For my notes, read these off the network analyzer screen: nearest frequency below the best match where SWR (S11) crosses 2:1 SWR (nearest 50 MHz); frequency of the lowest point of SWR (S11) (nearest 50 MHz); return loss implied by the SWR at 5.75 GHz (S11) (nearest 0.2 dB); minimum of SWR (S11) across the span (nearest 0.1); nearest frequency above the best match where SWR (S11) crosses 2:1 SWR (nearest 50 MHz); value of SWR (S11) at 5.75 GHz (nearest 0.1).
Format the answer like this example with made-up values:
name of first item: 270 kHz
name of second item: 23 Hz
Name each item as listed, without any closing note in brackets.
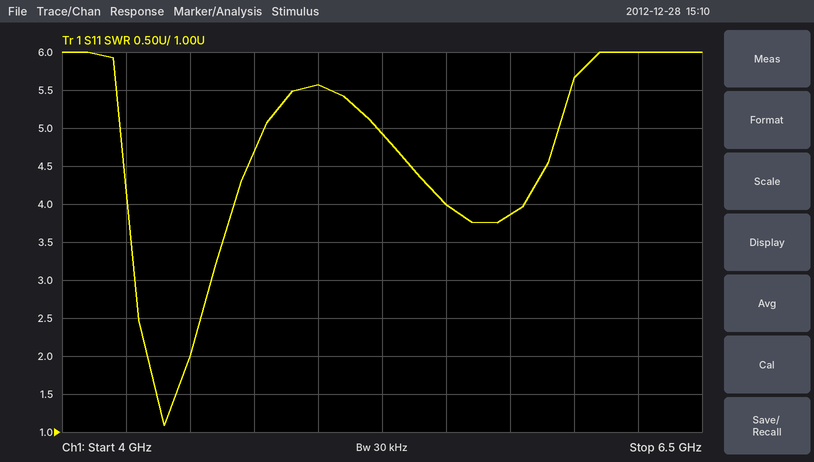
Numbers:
nearest frequency below the best match where SWR (S11) crosses 2:1 SWR: 4.35 GHz
frequency of the lowest point of SWR (S11): 4.40 GHz
return loss implied by the SWR at 5.75 GHz (S11): 4.6 dB
minimum of SWR (S11) across the span: 1.1
nearest frequency above the best match where SWR (S11) crosses 2:1 SWR: 4.50 GHz
value of SWR (S11) at 5.75 GHz: 3.9
